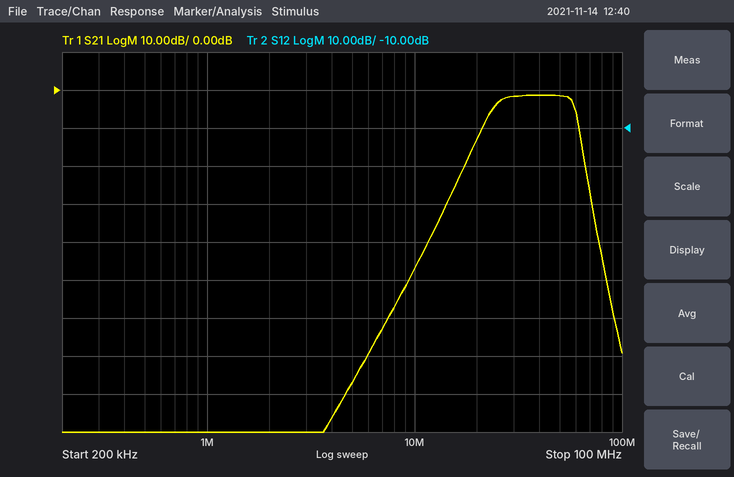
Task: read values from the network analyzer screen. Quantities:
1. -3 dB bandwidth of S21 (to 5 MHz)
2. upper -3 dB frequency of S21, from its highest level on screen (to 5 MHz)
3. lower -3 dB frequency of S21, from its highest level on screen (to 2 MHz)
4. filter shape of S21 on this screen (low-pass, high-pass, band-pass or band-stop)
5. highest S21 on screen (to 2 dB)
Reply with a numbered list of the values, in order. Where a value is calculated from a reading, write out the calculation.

1. 60 MHz − 24 MHz = 36 MHz
2. 60 MHz
3. 24 MHz
4. band-pass
5. -2 dB
